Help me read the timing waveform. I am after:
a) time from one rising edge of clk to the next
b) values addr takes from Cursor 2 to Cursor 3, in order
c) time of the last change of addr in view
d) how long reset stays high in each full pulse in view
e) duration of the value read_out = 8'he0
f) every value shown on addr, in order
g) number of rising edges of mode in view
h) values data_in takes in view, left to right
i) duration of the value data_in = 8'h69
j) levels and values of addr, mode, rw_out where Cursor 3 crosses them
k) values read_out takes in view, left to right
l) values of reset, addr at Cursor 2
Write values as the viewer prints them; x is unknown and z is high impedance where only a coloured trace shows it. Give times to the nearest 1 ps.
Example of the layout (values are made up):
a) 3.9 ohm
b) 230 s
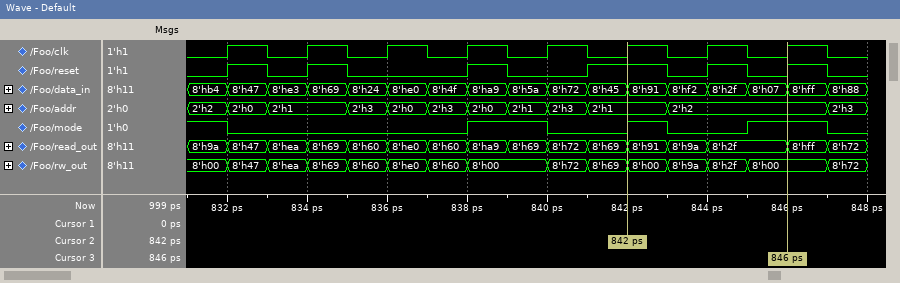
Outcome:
a) 2 ps
b) 2'h1, 2'h2
c) 847 ps
d) 1 ps, 1 ps, 1 ps, 2 ps, 1 ps, 1 ps
e) 1 ps
f) 2'h2, 2'h0, 2'h1, 2'h3, 2'h0, 2'h3, 2'h0, 2'h1, 2'h3, 2'h1, 2'h2, 2'h3
g) 3
h) 8'hb4, 8'h47, 8'he3, 8'h69, 8'h24, 8'he0, 8'h4f, 8'ha9, 8'h5a, 8'h72, 8'h45, 8'h91, 8'hf2, 8'h2f, 8'h07, 8'hff, 8'h88
i) 1 ps
j) addr=2'h2, mode=1, rw_out=8'h00
k) 8'h9a, 8'h47, 8'hea, 8'h69, 8'h60, 8'he0, 8'h60, 8'ha9, 8'h69, 8'h72, 8'h69, 8'h91, 8'h9a, 8'h2f, 8'hff, 8'h72
l) reset=1, addr=2'h1
